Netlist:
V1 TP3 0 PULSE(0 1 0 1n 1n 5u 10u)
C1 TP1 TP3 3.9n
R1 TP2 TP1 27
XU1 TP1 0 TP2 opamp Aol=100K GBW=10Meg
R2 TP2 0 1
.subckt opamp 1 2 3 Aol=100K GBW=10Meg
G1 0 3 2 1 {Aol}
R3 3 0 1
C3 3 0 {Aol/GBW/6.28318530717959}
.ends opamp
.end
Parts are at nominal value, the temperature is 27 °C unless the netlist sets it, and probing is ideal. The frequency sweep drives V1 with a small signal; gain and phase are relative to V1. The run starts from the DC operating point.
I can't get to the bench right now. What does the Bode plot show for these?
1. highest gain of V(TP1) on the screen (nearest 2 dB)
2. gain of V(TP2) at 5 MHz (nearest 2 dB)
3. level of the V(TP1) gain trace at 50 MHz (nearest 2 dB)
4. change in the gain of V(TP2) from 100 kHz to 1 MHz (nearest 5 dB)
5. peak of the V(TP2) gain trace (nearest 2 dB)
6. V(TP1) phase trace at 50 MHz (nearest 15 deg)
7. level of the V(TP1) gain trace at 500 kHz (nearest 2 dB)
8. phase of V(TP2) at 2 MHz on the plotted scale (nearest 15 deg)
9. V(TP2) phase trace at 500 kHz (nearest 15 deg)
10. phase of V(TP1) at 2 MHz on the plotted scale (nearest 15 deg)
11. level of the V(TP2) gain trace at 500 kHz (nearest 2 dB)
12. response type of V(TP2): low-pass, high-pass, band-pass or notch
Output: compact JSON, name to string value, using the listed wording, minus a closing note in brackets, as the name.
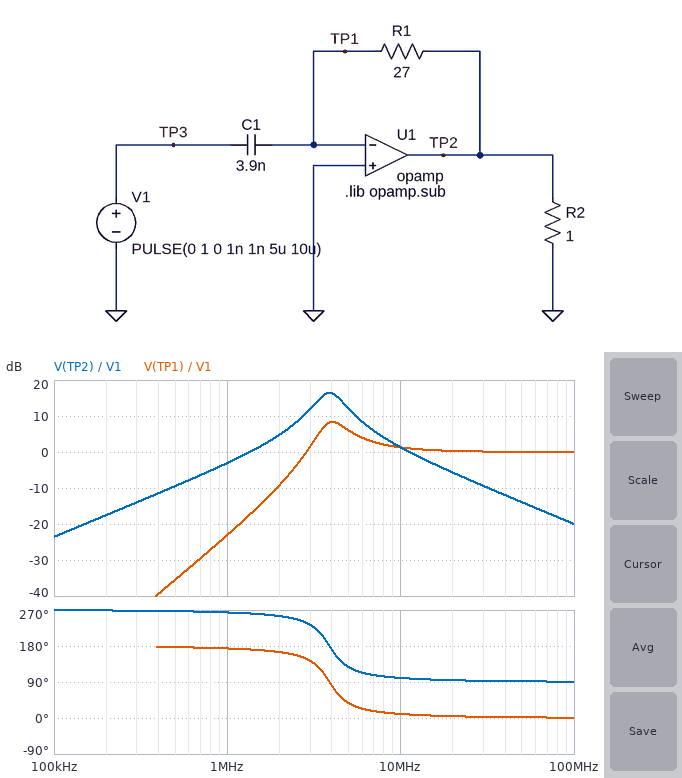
{"highest gain of V(TP1) on the screen": "8 dB", "gain of V(TP2) at 5 MHz": "12 dB", "level of the V(TP1) gain trace at 50 MHz": "0 dB", "change in the gain of V(TP2) from 100 kHz to 1 MHz": "20 dB", "peak of the V(TP2) gain trace": "16 dB", "V(TP1) phase trace at 50 MHz": "0 deg", "level of the V(TP1) gain trace at 500 kHz": "-36 dB", "phase of V(TP2) at 2 MHz on the plotted scale": "255 deg", "V(TP2) phase trace at 500 kHz": "270 deg", "phase of V(TP1) at 2 MHz on the plotted scale": "165 deg", "level of the V(TP2) gain trace at 500 kHz": "-10 dB", "response type of V(TP2): low-pass, high-pass, band-pass or notch": "band-pass"}
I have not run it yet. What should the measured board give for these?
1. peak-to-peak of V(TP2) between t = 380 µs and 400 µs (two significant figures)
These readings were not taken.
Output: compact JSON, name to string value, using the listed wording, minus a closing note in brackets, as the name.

{"peak-to-peak of V(TP2) between t = 380 µs and 400 µs": "3.9 V"}
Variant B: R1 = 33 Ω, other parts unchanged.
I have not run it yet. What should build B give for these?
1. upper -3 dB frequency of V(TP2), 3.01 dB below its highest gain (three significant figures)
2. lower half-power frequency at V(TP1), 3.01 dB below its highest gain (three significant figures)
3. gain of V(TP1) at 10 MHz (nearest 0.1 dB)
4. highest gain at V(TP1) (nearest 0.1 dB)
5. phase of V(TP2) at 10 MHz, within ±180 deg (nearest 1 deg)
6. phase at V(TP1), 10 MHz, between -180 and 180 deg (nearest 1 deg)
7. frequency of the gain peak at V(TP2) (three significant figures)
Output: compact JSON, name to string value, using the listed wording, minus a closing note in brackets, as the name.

{"upper -3 dB frequency of V(TP2), 3.01 dB below its highest gain": "4.19 MHz", "lower half-power frequency at V(TP1), 3.01 dB below its highest gain": "3.10 MHz", "gain of V(TP1) at 10 MHz": "1.1 dB", "highest gain at V(TP1)": "9.2 dB", "phase of V(TP2) at 10 MHz, within ±180 deg": "98 deg", "phase at V(TP1), 10 MHz, between -180 and 180 deg": "8 deg", "frequency of the gain peak at V(TP2)": "3.52 MHz"}
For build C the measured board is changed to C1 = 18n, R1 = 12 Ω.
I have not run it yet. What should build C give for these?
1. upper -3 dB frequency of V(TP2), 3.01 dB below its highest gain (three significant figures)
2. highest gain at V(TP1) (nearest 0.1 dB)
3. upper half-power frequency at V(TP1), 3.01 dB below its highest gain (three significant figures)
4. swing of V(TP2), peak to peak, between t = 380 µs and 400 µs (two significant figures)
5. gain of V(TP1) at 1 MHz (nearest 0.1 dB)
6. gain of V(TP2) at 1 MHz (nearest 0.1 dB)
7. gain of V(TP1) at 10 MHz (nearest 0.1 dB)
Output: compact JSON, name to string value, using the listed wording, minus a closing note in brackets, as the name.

{"upper -3 dB frequency of V(TP2), 3.01 dB below its highest gain": "3.11 MHz", "highest gain at V(TP1)": "11.4 dB", "upper half-power frequency at V(TP1), 3.01 dB below its highest gain": "3.26 MHz", "swing of V(TP2), peak to peak, between t = 380 µs and 400 µs": "6.1 V", "gain of V(TP1) at 1 MHz": "-16.1 dB", "gain of V(TP2) at 1 MHz": "3.9 dB", "gain of V(TP1) at 10 MHz": "0.6 dB"}
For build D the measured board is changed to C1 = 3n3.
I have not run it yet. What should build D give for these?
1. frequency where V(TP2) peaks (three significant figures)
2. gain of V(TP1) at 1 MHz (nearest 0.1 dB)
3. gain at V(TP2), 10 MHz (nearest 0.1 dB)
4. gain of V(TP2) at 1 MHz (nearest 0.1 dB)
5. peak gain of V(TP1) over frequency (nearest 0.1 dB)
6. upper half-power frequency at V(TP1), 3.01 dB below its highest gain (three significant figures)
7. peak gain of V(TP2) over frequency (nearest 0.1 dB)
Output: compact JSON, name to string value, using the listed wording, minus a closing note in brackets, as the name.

{"frequency where V(TP2) peaks": "4.23 MHz", "gain of V(TP1) at 1 MHz": "-24.6 dB", "gain at V(TP2), 10 MHz": "1.5 dB", "gain of V(TP2) at 1 MHz": "-4.6 dB", "peak gain of V(TP1) over frequency": "7.7 dB", "upper half-power frequency at V(TP1), 3.01 dB below its highest gain": "5.99 MHz", "peak gain of V(TP2) over frequency": "15.0 dB"}
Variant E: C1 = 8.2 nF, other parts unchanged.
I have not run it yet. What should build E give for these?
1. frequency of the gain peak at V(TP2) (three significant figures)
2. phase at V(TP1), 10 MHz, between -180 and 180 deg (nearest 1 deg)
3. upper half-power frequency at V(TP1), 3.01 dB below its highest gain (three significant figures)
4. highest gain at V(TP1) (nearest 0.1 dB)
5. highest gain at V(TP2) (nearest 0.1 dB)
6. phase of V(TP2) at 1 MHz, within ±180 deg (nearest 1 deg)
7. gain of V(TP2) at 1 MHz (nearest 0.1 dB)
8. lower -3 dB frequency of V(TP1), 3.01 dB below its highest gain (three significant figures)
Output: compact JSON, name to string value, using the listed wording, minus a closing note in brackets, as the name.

{"frequency of the gain peak at V(TP2)": "2.68 MHz", "phase at V(TP1), 10 MHz, between -180 and 180 deg": "4 deg", "upper half-power frequency at V(TP1), 3.01 dB below its highest gain": "3.21 MHz", "highest gain at V(TP1)": "11.5 dB", "highest gain at V(TP2)": "22.9 dB", "phase of V(TP2) at 1 MHz, within ±180 deg": "-97 deg", "gain of V(TP2) at 1 MHz": "4.1 dB", "lower -3 dB frequency of V(TP1), 3.01 dB below its highest gain": "2.42 MHz"}
